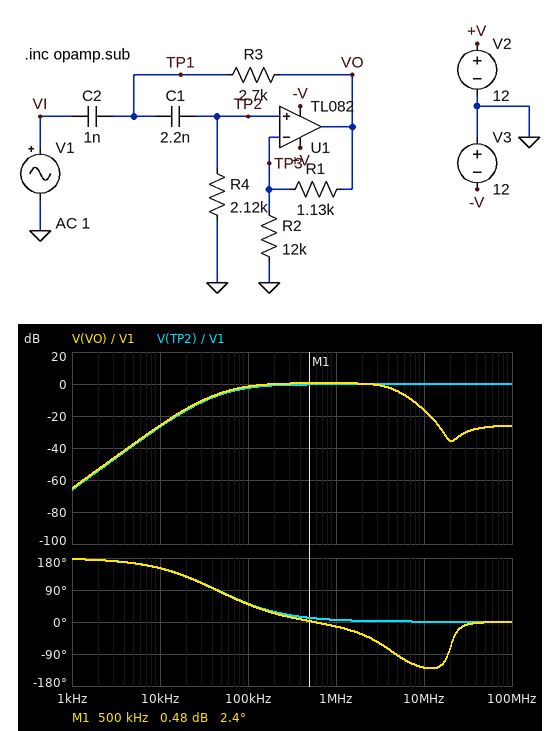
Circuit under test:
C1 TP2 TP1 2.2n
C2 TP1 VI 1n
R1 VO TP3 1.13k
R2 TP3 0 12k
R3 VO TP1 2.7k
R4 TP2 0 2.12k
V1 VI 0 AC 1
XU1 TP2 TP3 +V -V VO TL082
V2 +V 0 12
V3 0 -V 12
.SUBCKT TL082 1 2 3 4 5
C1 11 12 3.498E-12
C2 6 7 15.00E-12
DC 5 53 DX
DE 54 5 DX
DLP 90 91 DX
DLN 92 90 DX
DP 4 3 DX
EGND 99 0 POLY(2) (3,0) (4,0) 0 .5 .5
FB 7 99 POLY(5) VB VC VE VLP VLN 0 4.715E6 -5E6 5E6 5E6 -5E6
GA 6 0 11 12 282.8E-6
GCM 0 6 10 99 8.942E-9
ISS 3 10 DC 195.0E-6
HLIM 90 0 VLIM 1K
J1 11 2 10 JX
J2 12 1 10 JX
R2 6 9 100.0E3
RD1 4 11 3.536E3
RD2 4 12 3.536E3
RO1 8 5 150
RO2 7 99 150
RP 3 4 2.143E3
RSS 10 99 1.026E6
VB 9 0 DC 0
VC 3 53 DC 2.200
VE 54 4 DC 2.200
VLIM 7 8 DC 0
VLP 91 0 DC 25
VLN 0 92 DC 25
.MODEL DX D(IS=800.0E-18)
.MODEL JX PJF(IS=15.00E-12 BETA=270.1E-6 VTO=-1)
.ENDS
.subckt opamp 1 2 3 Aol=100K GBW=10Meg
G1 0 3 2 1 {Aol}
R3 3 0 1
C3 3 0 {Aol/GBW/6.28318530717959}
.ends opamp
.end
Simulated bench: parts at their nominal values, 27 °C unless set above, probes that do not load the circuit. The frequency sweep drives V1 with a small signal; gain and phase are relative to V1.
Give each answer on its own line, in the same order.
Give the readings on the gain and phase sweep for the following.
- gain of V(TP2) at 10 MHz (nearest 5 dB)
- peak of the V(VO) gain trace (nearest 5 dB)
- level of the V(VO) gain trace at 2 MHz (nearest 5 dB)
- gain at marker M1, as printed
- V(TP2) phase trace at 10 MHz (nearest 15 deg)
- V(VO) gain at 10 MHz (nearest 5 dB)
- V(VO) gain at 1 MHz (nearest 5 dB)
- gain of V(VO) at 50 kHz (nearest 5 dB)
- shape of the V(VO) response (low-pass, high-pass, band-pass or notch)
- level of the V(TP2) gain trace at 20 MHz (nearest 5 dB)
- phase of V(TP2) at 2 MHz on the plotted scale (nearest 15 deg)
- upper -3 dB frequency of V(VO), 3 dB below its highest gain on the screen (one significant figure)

0 dB
0 dB
0 dB
0.48 dB
0 deg
-15 dB
0 dB
-5 dB
band-pass
0 dB
0 deg
4 MHz
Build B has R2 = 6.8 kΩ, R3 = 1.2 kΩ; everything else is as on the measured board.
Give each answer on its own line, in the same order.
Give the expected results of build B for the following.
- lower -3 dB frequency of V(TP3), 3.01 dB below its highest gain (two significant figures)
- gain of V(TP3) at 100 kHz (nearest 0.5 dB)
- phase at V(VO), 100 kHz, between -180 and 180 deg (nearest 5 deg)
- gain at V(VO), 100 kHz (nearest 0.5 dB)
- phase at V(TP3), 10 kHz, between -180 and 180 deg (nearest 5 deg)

60 kHz
-0.5 dB
55 deg
1.0 dB
170 deg
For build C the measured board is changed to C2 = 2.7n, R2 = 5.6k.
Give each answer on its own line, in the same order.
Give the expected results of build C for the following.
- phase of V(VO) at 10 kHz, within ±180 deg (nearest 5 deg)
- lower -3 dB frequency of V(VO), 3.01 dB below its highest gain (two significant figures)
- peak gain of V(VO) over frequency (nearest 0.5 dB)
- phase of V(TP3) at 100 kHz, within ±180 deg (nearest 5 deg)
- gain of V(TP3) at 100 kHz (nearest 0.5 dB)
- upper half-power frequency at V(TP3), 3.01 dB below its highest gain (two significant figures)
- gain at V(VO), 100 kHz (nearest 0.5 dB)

140 deg
45 kHz
1.5 dB
30 deg
-1.0 dB
3.6 MHz
1.0 dB
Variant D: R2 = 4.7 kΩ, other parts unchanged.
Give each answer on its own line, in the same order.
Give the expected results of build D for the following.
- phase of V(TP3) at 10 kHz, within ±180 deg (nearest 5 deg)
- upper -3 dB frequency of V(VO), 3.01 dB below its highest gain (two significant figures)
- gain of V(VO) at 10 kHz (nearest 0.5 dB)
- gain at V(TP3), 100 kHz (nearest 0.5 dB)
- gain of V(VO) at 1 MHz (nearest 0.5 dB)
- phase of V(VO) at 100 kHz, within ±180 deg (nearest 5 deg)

155 deg
3.6 MHz
-24.5 dB
-2.0 dB
1.5 dB
45 deg
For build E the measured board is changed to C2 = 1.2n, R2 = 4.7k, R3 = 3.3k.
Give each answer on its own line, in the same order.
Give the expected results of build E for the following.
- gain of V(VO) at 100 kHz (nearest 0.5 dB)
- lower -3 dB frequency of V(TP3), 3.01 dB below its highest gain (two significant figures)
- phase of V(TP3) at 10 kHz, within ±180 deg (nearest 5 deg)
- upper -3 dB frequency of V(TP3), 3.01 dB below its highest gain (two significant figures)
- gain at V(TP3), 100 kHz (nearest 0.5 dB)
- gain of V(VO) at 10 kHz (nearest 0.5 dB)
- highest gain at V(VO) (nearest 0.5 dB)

0 dB
69 kHz
145 deg
3.6 MHz
-2.0 dB
-22.0 dB
1.5 dB
